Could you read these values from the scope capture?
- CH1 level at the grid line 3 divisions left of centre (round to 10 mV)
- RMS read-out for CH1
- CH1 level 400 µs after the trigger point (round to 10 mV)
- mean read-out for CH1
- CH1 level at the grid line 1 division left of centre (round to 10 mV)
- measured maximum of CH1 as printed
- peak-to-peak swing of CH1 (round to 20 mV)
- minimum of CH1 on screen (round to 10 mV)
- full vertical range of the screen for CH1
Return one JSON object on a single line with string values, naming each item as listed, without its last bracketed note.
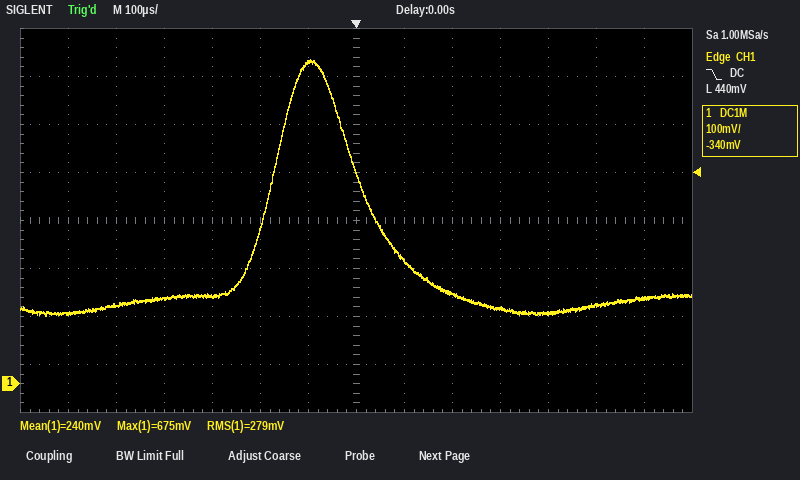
{"CH1 level at the grid line 3 divisions left of centre": "180 mV", "RMS read-out for CH1": "279 mV", "CH1 level 400 µs after the trigger point": "150 mV", "mean read-out for CH1": "240 mV", "CH1 level at the grid line 1 division left of centre": "670 mV", "measured maximum of CH1 as printed": "675 mV", "peak-to-peak swing of CH1": "540 mV", "minimum of CH1 on screen": "140 mV", "full vertical range of the screen for CH1": "800 mV"}
